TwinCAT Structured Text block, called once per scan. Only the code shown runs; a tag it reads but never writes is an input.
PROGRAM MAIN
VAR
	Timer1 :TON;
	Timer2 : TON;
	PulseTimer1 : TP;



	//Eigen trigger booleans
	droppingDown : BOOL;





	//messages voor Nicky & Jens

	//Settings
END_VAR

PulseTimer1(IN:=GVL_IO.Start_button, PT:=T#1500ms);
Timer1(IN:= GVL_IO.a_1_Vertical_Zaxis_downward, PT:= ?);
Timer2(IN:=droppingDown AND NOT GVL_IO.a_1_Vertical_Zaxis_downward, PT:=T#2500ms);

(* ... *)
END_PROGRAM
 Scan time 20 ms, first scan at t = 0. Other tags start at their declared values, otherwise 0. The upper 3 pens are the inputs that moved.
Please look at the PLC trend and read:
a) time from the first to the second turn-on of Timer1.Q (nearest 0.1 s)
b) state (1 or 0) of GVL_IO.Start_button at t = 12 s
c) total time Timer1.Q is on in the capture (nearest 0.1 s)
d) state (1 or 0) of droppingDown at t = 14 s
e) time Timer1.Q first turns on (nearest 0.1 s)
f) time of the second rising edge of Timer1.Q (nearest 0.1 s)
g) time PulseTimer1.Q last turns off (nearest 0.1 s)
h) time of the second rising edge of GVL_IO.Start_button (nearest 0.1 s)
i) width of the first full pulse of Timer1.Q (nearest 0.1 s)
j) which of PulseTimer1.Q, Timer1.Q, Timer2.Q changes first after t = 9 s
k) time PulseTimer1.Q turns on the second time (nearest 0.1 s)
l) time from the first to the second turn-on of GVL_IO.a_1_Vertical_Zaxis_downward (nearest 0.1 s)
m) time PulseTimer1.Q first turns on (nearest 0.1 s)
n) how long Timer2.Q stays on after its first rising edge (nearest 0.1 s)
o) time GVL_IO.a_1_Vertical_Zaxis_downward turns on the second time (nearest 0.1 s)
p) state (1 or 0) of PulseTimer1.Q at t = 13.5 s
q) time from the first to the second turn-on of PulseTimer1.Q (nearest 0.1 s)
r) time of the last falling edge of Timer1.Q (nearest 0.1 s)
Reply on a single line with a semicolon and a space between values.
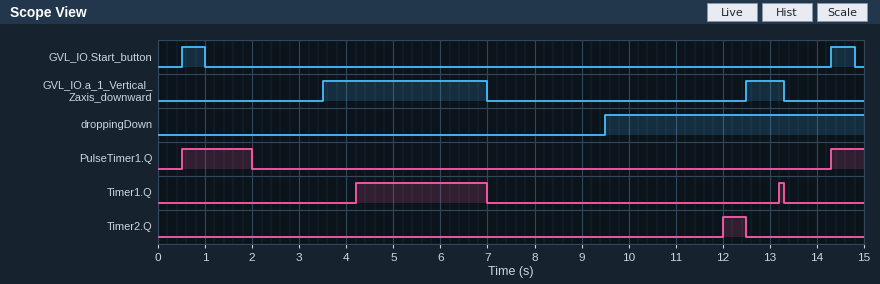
9.0 s; 0; 2.9 s; 1; 4.2 s; 13.2 s; 2.0 s; 14.3 s; 2.8 s; Timer2.Q; 14.3 s; 9.0 s; 0.5 s; 0.5 s; 12.5 s; 0; 13.8 s; 13.3 s
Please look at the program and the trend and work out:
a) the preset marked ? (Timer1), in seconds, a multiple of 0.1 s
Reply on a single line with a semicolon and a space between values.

0.7 s
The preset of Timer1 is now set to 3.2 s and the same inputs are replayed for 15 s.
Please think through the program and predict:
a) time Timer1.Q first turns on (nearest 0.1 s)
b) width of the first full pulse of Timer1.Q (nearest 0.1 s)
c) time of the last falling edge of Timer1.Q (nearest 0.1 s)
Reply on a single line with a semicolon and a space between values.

6.7 s; 0.3 s; 7.0 s
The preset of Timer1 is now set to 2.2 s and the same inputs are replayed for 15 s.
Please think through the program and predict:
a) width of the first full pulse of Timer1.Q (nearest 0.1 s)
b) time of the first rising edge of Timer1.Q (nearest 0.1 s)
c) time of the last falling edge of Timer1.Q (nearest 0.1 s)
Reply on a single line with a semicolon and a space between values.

1.3 s; 5.7 s; 7.0 s
